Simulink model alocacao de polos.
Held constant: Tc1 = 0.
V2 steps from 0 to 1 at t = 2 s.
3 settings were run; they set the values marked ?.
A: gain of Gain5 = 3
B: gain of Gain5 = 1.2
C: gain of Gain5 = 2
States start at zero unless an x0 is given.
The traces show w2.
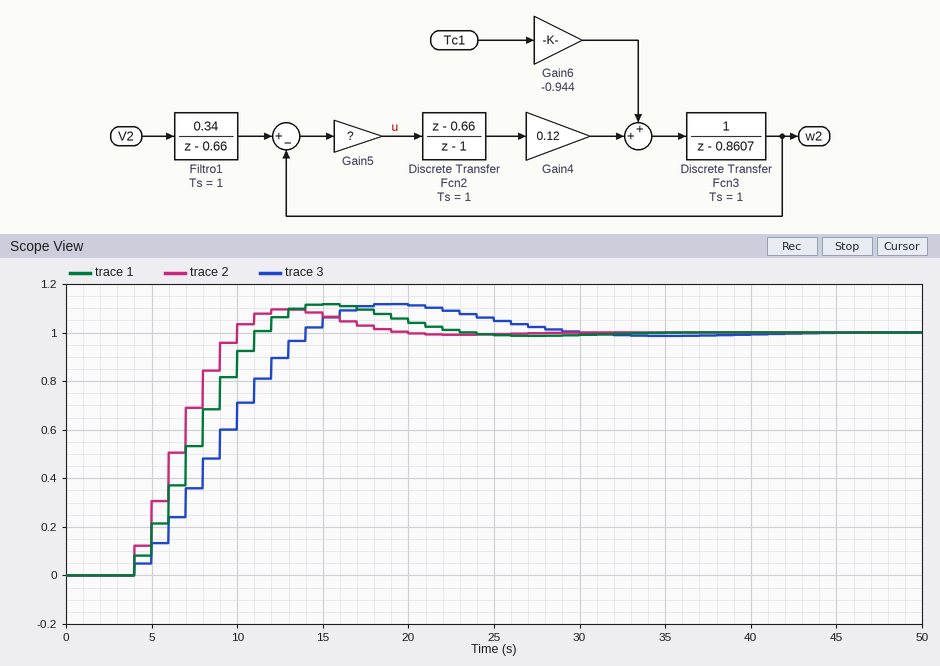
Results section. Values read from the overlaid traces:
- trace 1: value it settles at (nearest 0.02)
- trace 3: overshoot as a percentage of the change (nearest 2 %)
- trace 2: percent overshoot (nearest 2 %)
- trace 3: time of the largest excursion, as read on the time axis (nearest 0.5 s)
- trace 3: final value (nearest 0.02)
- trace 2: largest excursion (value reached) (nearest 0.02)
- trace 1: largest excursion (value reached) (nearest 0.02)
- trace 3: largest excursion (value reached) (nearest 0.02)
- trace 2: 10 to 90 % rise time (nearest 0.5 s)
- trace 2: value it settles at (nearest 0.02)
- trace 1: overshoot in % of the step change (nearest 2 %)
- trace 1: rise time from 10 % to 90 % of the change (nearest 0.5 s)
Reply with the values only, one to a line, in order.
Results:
1.00
12 %
10 %
19.0 s
1.00
1.10
1.12
1.12
5.0 s
1.00
12 %
5.0 s
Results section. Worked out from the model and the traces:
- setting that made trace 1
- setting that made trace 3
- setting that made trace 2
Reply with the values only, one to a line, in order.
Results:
C
B
A
